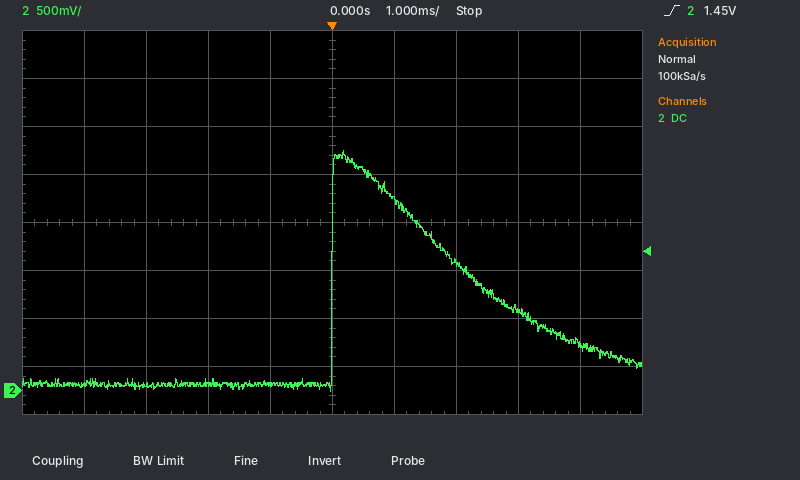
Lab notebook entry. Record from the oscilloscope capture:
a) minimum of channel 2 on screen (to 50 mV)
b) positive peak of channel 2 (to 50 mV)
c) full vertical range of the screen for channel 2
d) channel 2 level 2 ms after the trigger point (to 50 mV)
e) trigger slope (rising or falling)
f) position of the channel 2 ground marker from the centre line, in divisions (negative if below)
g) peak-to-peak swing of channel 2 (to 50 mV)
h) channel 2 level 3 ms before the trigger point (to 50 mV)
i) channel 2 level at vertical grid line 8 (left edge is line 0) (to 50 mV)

0 mV
2.50 V
4 V
1.35 V
rising
-3.5 div
2.50 V
50 mV
850 mV
